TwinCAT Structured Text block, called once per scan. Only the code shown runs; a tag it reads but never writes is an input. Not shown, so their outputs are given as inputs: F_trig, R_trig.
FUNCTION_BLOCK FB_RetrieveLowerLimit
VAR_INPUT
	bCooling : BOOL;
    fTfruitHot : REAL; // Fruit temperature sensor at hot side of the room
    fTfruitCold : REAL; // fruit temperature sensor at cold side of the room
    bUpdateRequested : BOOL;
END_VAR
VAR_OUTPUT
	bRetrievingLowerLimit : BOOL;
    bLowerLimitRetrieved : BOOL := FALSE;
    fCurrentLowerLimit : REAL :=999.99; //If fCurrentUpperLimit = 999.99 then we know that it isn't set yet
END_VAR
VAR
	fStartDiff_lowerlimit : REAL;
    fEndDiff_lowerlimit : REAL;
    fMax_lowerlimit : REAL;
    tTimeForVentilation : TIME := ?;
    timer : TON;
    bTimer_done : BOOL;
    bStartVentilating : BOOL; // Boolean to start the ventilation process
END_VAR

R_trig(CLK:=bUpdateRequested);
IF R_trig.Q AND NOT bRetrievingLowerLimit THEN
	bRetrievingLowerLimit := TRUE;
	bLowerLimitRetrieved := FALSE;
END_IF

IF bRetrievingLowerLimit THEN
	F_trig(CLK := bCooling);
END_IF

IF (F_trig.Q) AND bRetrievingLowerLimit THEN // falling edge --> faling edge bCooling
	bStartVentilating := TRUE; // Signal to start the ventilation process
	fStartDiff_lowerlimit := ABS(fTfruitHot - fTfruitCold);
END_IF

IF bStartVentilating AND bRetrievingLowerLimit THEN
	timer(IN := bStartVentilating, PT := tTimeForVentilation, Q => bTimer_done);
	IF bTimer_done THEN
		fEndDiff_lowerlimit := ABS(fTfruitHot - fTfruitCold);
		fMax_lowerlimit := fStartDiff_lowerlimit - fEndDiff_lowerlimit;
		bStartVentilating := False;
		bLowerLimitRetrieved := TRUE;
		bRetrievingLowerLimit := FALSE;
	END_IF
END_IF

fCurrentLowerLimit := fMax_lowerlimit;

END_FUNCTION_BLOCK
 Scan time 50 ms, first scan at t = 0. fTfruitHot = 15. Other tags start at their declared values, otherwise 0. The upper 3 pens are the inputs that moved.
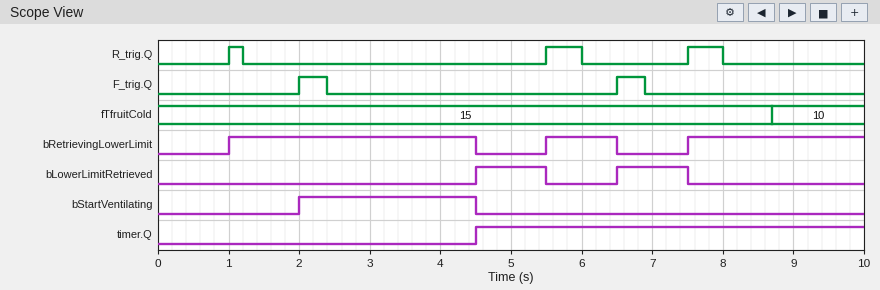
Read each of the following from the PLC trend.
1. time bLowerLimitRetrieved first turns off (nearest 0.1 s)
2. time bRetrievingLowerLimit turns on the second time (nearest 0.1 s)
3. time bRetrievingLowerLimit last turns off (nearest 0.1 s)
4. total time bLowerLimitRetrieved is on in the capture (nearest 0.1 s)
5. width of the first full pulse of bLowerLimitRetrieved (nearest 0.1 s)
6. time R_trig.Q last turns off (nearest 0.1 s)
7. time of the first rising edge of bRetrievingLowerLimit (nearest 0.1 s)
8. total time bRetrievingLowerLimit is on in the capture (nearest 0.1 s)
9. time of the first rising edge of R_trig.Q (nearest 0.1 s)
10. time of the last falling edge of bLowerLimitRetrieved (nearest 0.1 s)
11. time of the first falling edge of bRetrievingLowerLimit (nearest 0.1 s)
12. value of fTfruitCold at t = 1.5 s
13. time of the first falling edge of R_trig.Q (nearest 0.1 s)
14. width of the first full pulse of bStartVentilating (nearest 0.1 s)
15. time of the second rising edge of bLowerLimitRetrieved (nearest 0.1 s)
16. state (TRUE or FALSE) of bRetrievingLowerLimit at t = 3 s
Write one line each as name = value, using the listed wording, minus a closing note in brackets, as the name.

time bLowerLimitRetrieved first turns off = 5.5 s
time bRetrievingLowerLimit turns on the second time = 5.5 s
time bRetrievingLowerLimit last turns off = 6.5 s
total time bLowerLimitRetrieved is on in the capture = 2.0 s
width of the first full pulse of bLowerLimitRetrieved = 1.0 s
time R_trig.Q last turns off = 8.0 s
time of the first rising edge of bRetrievingLowerLimit = 1.0 s
total time bRetrievingLowerLimit is on in the capture = 7.0 s
time of the first rising edge of R_trig.Q = 1.0 s
time of the last falling edge of bLowerLimitRetrieved = 7.5 s
time of the first falling edge of bRetrievingLowerLimit = 4.5 s
value of fTfruitCold at t = 1.5 s = 15
time of the first falling edge of R_trig.Q = 1.2 s
width of the first full pulse of bStartVentilating = 2.5 s
time of the second rising edge of bLowerLimitRetrieved = 6.5 s
state (TRUE or FALSE) of bRetrievingLowerLimit at t = 3 s = TRUE
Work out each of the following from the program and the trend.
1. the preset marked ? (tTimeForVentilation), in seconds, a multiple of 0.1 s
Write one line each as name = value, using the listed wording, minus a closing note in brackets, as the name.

the preset marked ? (tTimeForVentilation), in seconds, a multiple of 0.1 s = 2.5 s
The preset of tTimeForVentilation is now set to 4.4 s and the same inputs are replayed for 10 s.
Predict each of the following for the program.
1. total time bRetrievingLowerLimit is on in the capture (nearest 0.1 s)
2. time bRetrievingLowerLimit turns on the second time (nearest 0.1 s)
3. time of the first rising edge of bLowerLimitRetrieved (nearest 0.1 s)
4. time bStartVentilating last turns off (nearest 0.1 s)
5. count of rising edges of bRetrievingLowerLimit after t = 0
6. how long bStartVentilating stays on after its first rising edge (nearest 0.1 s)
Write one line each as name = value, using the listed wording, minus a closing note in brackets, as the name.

total time bRetrievingLowerLimit is on in the capture = 7.9 s
time bRetrievingLowerLimit turns on the second time = 7.5 s
time of the first rising edge of bLowerLimitRetrieved = 6.4 s
time bStartVentilating last turns off = 6.4 s
count of rising edges of bRetrievingLowerLimit after t = 0 = 2
how long bStartVentilating stays on after its first rising edge = 4.4 s
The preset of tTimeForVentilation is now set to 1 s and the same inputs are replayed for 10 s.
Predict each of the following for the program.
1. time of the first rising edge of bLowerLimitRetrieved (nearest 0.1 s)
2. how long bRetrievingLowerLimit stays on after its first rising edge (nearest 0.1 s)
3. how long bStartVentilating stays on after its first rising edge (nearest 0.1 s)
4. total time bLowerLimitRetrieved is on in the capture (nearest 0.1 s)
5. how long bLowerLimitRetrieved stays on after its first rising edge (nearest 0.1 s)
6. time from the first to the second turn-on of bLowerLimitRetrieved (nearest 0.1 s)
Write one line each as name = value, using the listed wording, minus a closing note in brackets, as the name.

time of the first rising edge of bLowerLimitRetrieved = 3.0 s
how long bRetrievingLowerLimit stays on after its first rising edge = 2.0 s
how long bStartVentilating stays on after its first rising edge = 1.0 s
total time bLowerLimitRetrieved is on in the capture = 3.5 s
how long bLowerLimitRetrieved stays on after its first rising edge = 2.5 s
time from the first to the second turn-on of bLowerLimitRetrieved = 3.5 s
